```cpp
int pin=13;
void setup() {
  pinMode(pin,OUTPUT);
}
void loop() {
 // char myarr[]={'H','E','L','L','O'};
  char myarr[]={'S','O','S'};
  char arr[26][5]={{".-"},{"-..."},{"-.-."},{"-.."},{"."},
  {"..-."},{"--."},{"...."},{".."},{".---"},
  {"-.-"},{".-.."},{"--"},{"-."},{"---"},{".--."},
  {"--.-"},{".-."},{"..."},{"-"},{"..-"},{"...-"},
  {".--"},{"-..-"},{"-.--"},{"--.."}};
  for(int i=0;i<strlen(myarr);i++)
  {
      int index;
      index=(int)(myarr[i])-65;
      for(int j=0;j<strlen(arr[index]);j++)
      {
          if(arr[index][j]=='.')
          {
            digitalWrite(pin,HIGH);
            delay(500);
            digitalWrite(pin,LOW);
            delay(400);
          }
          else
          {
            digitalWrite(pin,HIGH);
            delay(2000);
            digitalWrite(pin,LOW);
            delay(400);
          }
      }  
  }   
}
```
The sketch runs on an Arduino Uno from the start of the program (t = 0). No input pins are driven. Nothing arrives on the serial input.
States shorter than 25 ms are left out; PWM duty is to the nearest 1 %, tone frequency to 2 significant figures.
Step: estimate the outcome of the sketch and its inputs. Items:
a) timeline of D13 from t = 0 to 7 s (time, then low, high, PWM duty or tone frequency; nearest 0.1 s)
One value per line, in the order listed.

0 s high; 0.5 s low; 0.9 s high; 1.4 s low; 1.8 s high; 2.3 s low; 2.7 s high; 4.7 s low; 5.1 s high
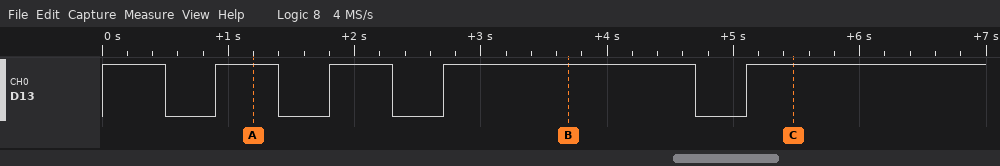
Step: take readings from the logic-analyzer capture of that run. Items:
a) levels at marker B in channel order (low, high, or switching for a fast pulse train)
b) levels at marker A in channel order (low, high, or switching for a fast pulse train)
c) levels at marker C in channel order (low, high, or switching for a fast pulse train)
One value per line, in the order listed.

D13 high
D13 high
D13 high
